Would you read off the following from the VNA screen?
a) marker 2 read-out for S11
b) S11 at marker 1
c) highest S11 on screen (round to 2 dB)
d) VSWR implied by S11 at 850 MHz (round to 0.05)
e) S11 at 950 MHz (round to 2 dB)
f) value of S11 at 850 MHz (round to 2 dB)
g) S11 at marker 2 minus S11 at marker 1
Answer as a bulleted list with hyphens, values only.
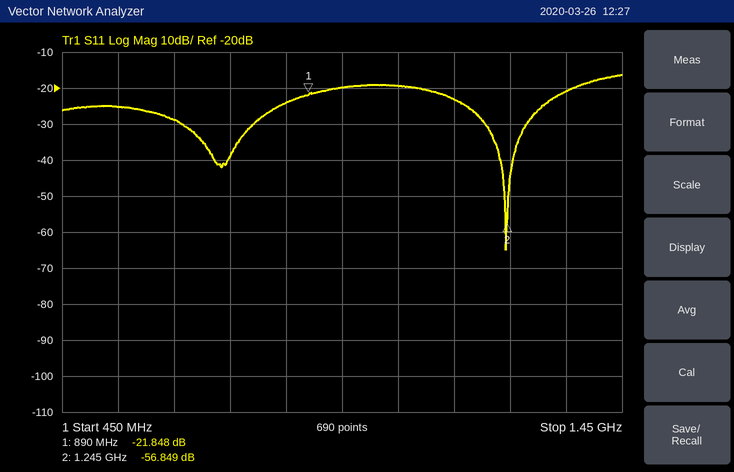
- -56.849 dB
- -21.848 dB
- -16 dB
- 1.15
- -20 dB
- -24 dB
- -35.001 dB
